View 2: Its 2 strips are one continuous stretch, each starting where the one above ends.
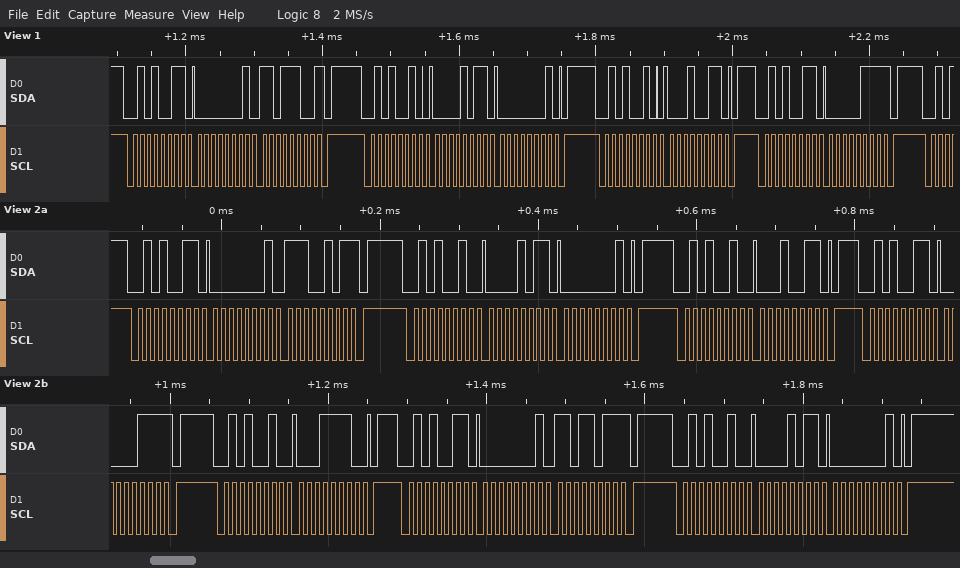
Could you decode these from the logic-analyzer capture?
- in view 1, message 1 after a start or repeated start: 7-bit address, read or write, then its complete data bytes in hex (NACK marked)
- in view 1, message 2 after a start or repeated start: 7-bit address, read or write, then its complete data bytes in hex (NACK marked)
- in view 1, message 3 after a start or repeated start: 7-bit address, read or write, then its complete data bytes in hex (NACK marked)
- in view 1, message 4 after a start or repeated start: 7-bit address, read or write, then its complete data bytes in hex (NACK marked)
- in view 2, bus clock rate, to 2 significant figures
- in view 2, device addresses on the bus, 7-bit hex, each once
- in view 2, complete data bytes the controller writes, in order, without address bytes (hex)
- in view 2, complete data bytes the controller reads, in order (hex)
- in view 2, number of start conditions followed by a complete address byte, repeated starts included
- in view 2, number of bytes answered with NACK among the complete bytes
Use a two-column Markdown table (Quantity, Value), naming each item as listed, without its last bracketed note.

| Quantity | Value |
|---|---|
| in view 1, message 1 after a start or repeated start: 7-bit address, read or write, then its complete data bytes in hex | 0x29 read: 01 DC NACK |
| in view 1, message 2 after a start or repeated start: 7-bit address, read or write, then its complete data bytes in hex | 0x29 write: 0B 01 |
| in view 1, message 3 after a start or repeated start: 7-bit address, read or write, then its complete data bytes in hex | 0x29 write: 13 |
| in view 1, message 4 after a start or repeated start: 7-bit address, read or write, then its complete data bytes in hex | 0x29 read: 07 NACK |
| in view 2, bus clock rate, to 2 significant figures | 100 kHz |
| in view 2, device addresses on the bus, 7-bit hex, each once | 0x29 |
| in view 2, complete data bytes the controller writes, in order, without address bytes | 0B 01 13 1E 0B 01 |
| in view 2, complete data bytes the controller reads, in order | 01 E5 07 01 DB |
| in view 2, number of start conditions followed by a complete address byte, repeated starts included | 7 |
| in view 2, number of bytes answered with NACK among the complete bytes | 3 |
